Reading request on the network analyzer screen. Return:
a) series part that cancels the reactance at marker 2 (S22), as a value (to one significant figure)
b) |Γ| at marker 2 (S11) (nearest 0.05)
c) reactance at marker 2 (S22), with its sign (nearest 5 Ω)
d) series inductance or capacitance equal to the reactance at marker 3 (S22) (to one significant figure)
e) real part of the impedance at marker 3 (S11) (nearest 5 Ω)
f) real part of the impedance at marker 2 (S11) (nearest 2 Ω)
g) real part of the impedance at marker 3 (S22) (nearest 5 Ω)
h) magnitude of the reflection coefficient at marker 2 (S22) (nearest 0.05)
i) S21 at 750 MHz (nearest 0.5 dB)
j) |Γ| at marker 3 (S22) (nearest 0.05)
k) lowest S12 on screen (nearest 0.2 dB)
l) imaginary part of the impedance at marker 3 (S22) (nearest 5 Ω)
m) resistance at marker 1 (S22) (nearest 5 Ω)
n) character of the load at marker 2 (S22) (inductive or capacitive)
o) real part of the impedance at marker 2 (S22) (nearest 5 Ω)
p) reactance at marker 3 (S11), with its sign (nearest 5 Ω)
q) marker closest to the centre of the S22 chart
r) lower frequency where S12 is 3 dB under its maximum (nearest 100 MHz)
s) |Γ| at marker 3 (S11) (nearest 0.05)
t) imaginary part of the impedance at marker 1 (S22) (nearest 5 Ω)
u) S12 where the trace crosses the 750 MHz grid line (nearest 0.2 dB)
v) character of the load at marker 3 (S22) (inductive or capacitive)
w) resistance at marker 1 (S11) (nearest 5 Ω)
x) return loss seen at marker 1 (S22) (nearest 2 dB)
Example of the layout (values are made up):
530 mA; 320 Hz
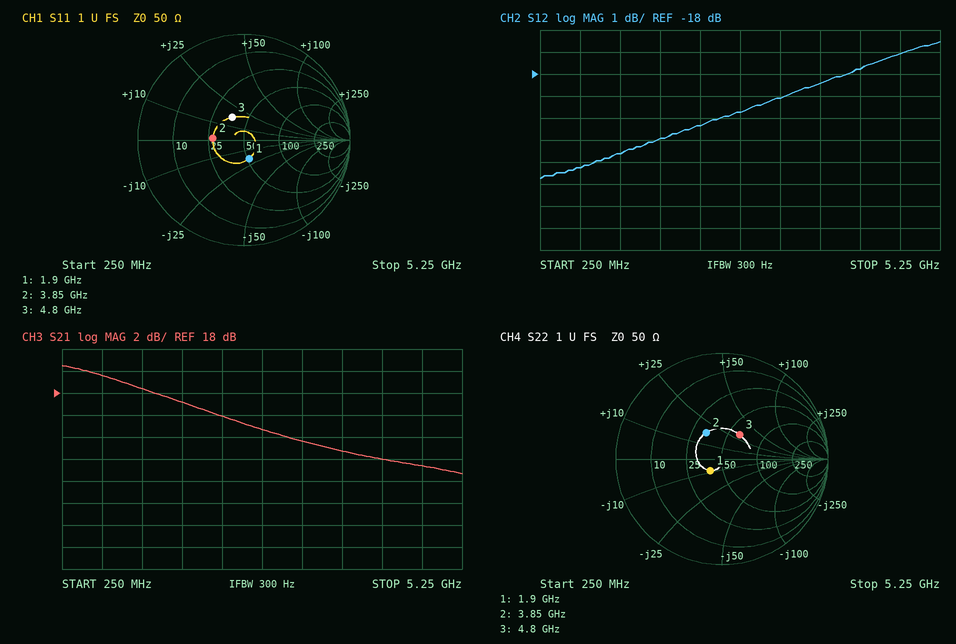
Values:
2 pF; 0.30; +20 Ω; 1 nH; 35 Ω; 28 Ω; 60 Ω; 0.30; 19.5 dB; 0.30; -22.8 dB; +30 Ω; 40 Ω; inductive; 35 Ω; +15 Ω; marker 1; 2.9 GHz; 0.25; -10 Ω; -22.2 dB; inductive; 50 Ω; 16 dB
